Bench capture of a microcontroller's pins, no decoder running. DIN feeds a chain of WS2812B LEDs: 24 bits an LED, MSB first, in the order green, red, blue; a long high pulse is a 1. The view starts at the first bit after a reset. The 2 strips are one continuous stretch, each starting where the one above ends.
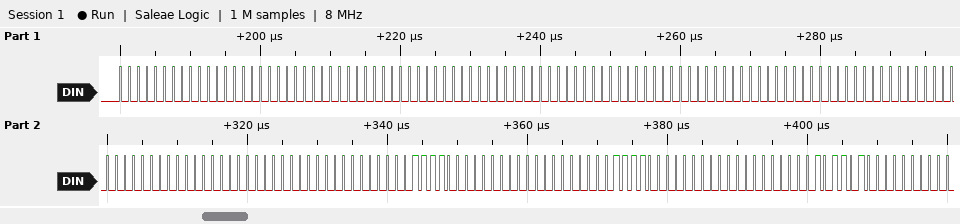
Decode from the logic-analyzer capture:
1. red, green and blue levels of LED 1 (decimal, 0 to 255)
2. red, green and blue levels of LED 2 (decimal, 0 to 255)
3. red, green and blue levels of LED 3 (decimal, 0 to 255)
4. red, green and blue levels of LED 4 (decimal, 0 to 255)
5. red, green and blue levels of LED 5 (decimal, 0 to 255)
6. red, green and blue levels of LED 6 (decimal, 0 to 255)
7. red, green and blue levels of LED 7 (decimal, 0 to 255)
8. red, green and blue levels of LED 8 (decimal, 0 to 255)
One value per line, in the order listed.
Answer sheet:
0, 0, 0
0, 0, 0
0, 0, 0
0, 0, 0
0, 0, 0
30, 0, 0
60, 0, 0
90, 0, 0
